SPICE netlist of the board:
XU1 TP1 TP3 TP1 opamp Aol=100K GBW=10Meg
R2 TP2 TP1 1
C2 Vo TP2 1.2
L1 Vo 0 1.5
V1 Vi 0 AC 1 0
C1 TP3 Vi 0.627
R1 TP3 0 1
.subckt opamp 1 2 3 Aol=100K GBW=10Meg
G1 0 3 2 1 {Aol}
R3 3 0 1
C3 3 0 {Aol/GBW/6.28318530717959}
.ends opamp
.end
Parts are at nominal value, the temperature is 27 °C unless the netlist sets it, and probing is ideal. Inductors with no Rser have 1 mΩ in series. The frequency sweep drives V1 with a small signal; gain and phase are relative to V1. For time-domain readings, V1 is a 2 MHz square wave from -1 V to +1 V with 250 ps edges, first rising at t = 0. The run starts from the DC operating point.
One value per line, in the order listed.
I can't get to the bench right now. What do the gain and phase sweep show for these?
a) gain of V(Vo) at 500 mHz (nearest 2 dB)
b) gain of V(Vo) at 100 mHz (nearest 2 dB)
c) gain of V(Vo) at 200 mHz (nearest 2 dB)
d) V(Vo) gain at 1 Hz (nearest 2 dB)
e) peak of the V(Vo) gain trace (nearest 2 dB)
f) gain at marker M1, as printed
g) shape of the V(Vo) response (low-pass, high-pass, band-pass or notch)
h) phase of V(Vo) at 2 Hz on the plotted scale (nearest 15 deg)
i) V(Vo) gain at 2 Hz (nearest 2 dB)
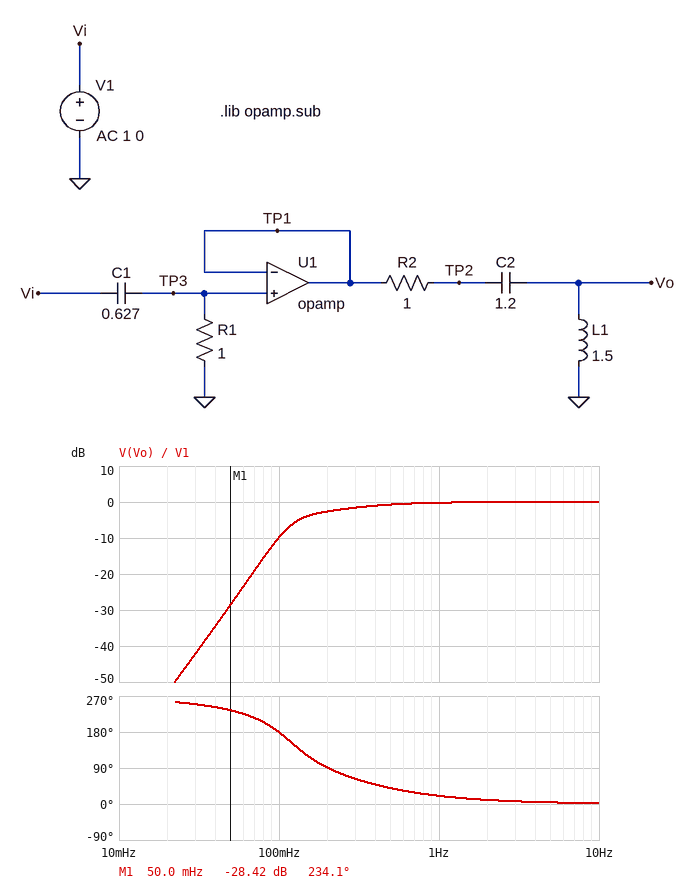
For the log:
0 dB
-10 dB
-2 dB
0 dB
0 dB
-28.42 dB
high-pass
15 deg
0 dB
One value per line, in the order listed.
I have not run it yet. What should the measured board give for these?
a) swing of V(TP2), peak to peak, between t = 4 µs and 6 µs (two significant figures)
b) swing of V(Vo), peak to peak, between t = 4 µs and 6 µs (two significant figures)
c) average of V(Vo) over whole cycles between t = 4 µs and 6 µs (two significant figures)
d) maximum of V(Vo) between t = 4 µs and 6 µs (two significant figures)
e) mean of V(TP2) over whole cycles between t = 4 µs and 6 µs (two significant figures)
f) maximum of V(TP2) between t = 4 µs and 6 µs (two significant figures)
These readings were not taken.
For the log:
2.0 V
2.0 V
1.0 V
2.0 V
1.0 V
2.0 V
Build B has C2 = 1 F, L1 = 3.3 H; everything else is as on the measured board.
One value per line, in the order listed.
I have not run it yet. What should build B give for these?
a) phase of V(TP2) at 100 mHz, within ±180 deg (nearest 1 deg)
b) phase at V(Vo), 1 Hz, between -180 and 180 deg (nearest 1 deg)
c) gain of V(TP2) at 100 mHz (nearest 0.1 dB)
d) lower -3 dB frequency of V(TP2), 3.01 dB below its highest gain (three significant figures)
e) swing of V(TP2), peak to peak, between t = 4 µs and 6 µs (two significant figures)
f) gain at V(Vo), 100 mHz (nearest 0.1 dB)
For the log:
133 deg
17 deg
-16.0 dB
265 mHz
2.0 V
-3.3 dB
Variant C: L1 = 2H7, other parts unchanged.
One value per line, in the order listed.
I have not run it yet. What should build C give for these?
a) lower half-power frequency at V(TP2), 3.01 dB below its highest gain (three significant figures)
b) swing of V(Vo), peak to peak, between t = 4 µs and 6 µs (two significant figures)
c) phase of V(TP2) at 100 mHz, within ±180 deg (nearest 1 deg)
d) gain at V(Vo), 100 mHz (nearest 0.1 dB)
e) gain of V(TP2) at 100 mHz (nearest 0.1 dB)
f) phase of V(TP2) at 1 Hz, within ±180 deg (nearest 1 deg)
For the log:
270 mHz
2.0 V
138 deg
-4.7 dB
-17.9 dB
18 deg
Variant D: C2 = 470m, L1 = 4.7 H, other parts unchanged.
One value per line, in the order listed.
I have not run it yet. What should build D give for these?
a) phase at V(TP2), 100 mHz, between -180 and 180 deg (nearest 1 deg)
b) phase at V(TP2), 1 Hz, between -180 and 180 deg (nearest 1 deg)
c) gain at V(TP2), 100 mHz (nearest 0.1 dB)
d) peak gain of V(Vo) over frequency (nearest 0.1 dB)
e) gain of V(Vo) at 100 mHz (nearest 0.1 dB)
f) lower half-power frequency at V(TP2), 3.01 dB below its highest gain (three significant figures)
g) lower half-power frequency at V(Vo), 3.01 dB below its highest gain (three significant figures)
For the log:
2 deg
16 deg
-16.7 dB
2.2 dB
-0.1 dB
260 mHz
98.0 mHz
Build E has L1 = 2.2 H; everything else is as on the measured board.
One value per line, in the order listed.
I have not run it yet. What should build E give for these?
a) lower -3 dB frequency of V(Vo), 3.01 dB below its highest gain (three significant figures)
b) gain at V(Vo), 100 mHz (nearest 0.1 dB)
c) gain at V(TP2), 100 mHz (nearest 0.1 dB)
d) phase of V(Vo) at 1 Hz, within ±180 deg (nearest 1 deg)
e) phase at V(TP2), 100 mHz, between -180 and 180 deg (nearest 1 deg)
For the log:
174 mHz
-5.9 dB
-33.8 dB
18 deg
154 deg
